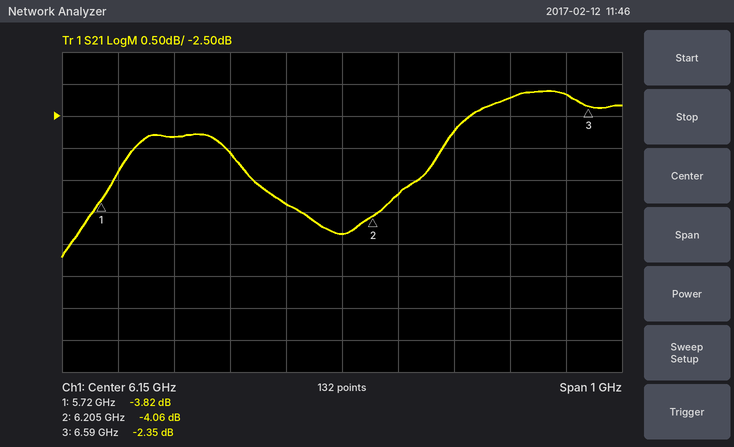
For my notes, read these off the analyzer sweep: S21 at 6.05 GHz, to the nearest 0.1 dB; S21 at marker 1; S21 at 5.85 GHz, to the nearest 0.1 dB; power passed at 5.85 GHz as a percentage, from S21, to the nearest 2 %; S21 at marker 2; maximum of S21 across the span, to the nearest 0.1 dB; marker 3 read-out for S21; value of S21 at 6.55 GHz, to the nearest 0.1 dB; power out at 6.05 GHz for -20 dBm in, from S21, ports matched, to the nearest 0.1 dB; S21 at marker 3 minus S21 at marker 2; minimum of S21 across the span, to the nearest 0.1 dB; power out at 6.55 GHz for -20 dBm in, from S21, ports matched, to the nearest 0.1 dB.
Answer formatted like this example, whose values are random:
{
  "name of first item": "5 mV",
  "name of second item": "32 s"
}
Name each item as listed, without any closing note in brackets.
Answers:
{
  "S21 at 6.05 GHz, to the nearest 0.1 dB": "-3.9 dB",
  "S21 at marker 1": "-3.82 dB",
  "S21 at 5.85 GHz, to the nearest 0.1 dB": "-2.8 dB",
  "power passed at 5.85 GHz as a percentage, from S21, to the nearest 2 %": "52 %",
  "S21 at marker 2": "-4.06 dB",
  "maximum of S21 across the span, to the nearest 0.1 dB": "-2.1 dB",
  "marker 3 read-out for S21": "-2.35 dB",
  "value of S21 at 6.55 GHz, to the nearest 0.1 dB": "-2.2 dB",
  "power out at 6.05 GHz for -20 dBm in, from S21, ports matched, to the nearest 0.1 dB": "-23.9 dBm",
  "S21 at marker 3 minus S21 at marker 2": "1.71 dB",
  "minimum of S21 across the span, to the nearest 0.1 dB": "-4.7 dB",
  "power out at 6.55 GHz for -20 dBm in, from S21, ports matched, to the nearest 0.1 dB": "-22.2 dBm"
}
